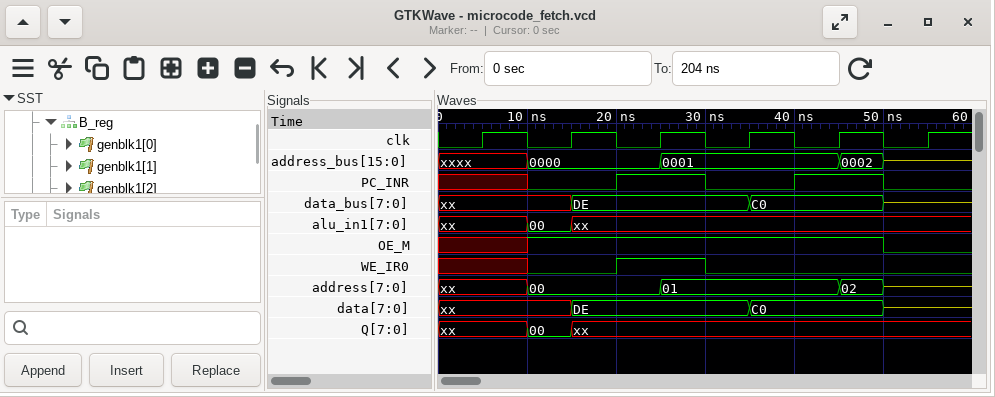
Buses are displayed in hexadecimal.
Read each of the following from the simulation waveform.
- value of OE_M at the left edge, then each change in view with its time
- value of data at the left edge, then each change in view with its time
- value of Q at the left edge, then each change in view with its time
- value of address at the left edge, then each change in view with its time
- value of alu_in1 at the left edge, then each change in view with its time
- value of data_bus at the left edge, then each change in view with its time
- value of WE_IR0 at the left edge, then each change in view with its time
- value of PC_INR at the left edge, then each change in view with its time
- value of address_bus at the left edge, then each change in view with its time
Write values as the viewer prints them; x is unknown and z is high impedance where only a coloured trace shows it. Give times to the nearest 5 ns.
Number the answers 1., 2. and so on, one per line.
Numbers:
1. x, 1 at 10 ns, 0 at 50 ns
2. xx, DE at 15 ns, C0 at 35 ns, z at 50 ns
3. xx, 00 at 10 ns, xx at 15 ns
4. xx, 00 at 10 ns, 01 at 25 ns, 02 at 45 ns, z at 50 ns
5. xx, 00 at 10 ns, xx at 15 ns
6. xx, DE at 15 ns, C0 at 35 ns, z at 50 ns
7. x, 0 at 10 ns, 1 at 20 ns, 0 at 30 ns
8. x, 0 at 10 ns, 1 at 20 ns, 0 at 30 ns, 1 at 40 ns, 0 at 50 ns
9. xxxx, 0000 at 10 ns, 0001 at 25 ns, 0002 at 45 ns, z at 50 ns
